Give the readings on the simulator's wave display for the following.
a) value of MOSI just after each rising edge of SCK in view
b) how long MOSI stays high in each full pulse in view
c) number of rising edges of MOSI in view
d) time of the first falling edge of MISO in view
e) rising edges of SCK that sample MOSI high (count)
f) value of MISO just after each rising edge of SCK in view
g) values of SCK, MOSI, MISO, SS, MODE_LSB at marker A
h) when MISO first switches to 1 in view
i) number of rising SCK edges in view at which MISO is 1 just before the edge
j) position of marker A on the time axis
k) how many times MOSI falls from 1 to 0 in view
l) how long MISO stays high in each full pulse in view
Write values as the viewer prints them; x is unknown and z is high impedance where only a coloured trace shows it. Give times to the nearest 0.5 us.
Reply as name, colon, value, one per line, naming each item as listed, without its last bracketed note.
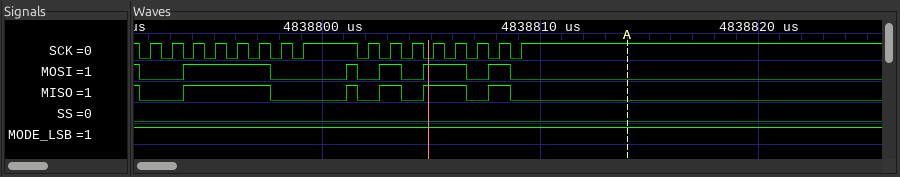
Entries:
value of MOSI just after each rising edge of SCK in view: 0 0 1 1 1 1 0 0 0 1 0 1 1 0 1 0
how long MOSI stays high in each full pulse in view: 4 us, 0.5 us, 1 us, 2 us, 1 us
number of rising edges of MOSI in view: 5
time of the first falling edge of MISO in view: 4838791.5 us
rising edges of SCK that sample MOSI high: 8
value of MISO just after each rising edge of SCK in view: 0 0 1 1 1 1 0 0 0 1 0 1 1 0 1 0
values of SCK, MOSI, MISO, SS, MODE_LSB at marker A: SCK=1, MOSI=0, MISO=0, SS=0, MODE_LSB=1
when MISO first switches to 1 in view: 4838793.5 us
number of rising SCK edges in view at which MISO is 1 just before the edge: 8
position of marker A on the time axis: 4838814 us
how many times MOSI falls from 1 to 0 in view: 6
how long MISO stays high in each full pulse in view: 4 us, 0.5 us, 1 us, 2 us, 1 us
